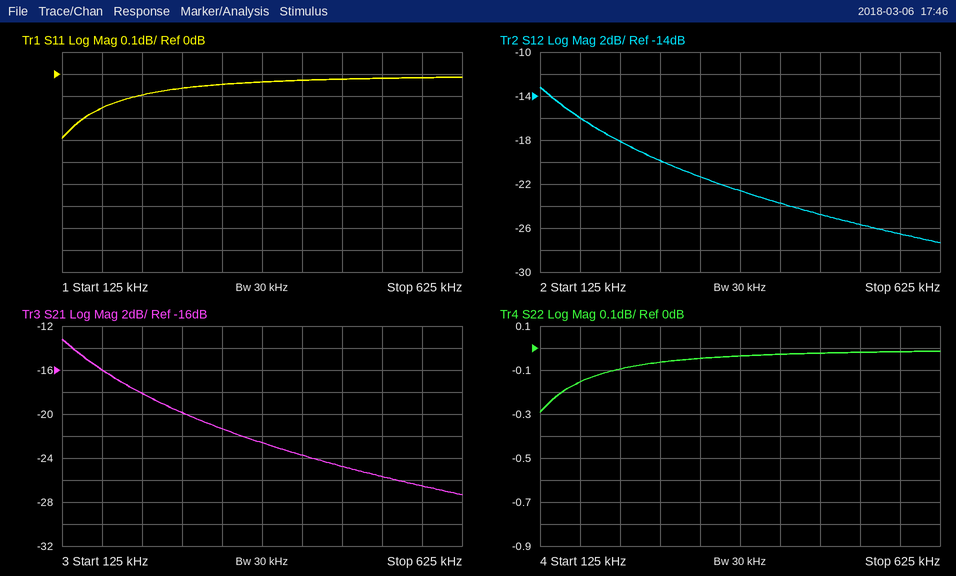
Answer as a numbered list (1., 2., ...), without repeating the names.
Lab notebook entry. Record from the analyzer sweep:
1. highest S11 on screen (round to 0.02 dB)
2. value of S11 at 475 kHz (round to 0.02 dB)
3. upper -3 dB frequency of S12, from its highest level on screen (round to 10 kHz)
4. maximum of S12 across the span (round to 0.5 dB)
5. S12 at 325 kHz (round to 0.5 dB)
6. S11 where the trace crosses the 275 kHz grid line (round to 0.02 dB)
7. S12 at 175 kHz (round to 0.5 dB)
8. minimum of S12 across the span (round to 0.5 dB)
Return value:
1. -0.02 dB
2. -0.02 dB
3. 180 kHz
4. -13.0 dB
5. -21.5 dB
6. -0.06 dB
7. -16.0 dB
8. -27.5 dB
